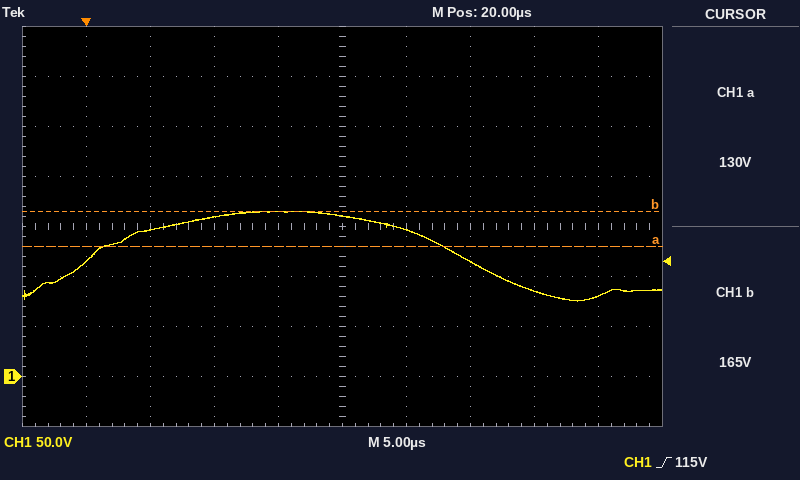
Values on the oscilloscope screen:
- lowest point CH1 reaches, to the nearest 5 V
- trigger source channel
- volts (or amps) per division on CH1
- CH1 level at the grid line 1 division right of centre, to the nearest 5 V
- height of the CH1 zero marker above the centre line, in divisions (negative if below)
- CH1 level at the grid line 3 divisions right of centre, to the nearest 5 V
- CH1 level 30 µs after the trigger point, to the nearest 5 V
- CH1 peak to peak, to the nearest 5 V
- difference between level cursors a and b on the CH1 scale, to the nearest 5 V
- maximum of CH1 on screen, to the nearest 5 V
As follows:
75 V
CH1
50 V
145 V
-3.0 div
85 V
115 V
90 V
35 V
165 V
